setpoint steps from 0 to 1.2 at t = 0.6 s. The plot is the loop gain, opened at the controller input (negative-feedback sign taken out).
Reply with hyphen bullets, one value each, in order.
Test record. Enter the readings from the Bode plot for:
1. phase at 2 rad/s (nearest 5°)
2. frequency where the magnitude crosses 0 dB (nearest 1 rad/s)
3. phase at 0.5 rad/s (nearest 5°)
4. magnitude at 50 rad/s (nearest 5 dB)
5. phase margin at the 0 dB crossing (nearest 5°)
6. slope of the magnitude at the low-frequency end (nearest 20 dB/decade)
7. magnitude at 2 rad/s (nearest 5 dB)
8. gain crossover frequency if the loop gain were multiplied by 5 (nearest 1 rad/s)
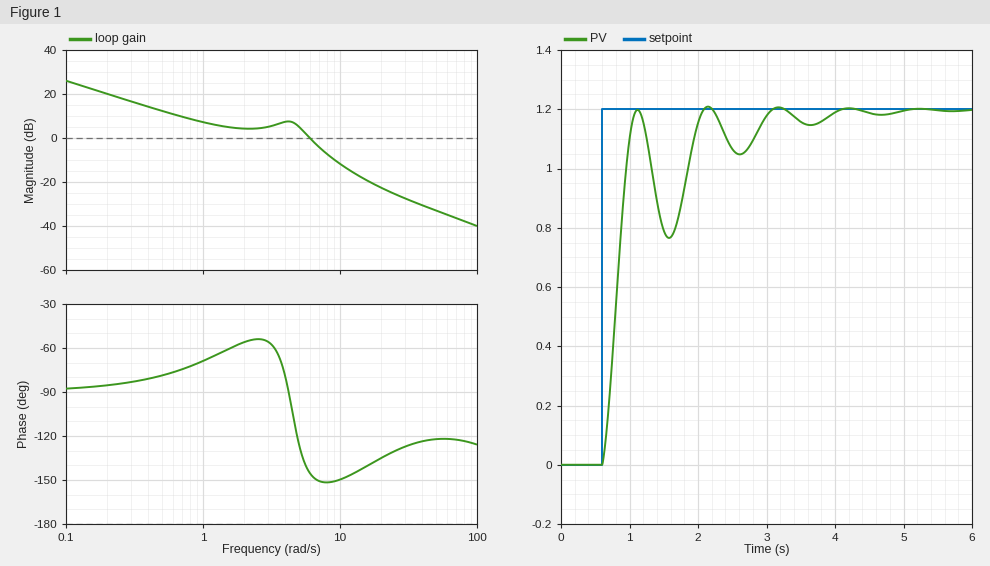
- -55°
- 6 rad/s
- -80°
- -35 dB
- 35°
- -20 dB/decade
- 5 dB
- 11 rad/s
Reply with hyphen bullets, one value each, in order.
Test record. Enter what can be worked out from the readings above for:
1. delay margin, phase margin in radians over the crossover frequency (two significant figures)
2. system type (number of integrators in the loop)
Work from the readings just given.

- 0.10 s
- 1
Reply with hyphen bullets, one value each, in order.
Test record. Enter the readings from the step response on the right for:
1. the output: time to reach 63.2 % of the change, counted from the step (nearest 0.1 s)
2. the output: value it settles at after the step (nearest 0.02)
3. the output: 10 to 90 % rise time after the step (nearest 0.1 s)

- 0.3 s
- 1.20
- 0.3 s
